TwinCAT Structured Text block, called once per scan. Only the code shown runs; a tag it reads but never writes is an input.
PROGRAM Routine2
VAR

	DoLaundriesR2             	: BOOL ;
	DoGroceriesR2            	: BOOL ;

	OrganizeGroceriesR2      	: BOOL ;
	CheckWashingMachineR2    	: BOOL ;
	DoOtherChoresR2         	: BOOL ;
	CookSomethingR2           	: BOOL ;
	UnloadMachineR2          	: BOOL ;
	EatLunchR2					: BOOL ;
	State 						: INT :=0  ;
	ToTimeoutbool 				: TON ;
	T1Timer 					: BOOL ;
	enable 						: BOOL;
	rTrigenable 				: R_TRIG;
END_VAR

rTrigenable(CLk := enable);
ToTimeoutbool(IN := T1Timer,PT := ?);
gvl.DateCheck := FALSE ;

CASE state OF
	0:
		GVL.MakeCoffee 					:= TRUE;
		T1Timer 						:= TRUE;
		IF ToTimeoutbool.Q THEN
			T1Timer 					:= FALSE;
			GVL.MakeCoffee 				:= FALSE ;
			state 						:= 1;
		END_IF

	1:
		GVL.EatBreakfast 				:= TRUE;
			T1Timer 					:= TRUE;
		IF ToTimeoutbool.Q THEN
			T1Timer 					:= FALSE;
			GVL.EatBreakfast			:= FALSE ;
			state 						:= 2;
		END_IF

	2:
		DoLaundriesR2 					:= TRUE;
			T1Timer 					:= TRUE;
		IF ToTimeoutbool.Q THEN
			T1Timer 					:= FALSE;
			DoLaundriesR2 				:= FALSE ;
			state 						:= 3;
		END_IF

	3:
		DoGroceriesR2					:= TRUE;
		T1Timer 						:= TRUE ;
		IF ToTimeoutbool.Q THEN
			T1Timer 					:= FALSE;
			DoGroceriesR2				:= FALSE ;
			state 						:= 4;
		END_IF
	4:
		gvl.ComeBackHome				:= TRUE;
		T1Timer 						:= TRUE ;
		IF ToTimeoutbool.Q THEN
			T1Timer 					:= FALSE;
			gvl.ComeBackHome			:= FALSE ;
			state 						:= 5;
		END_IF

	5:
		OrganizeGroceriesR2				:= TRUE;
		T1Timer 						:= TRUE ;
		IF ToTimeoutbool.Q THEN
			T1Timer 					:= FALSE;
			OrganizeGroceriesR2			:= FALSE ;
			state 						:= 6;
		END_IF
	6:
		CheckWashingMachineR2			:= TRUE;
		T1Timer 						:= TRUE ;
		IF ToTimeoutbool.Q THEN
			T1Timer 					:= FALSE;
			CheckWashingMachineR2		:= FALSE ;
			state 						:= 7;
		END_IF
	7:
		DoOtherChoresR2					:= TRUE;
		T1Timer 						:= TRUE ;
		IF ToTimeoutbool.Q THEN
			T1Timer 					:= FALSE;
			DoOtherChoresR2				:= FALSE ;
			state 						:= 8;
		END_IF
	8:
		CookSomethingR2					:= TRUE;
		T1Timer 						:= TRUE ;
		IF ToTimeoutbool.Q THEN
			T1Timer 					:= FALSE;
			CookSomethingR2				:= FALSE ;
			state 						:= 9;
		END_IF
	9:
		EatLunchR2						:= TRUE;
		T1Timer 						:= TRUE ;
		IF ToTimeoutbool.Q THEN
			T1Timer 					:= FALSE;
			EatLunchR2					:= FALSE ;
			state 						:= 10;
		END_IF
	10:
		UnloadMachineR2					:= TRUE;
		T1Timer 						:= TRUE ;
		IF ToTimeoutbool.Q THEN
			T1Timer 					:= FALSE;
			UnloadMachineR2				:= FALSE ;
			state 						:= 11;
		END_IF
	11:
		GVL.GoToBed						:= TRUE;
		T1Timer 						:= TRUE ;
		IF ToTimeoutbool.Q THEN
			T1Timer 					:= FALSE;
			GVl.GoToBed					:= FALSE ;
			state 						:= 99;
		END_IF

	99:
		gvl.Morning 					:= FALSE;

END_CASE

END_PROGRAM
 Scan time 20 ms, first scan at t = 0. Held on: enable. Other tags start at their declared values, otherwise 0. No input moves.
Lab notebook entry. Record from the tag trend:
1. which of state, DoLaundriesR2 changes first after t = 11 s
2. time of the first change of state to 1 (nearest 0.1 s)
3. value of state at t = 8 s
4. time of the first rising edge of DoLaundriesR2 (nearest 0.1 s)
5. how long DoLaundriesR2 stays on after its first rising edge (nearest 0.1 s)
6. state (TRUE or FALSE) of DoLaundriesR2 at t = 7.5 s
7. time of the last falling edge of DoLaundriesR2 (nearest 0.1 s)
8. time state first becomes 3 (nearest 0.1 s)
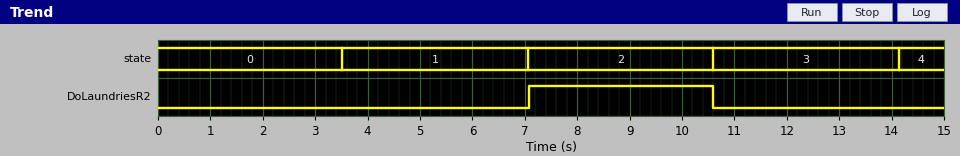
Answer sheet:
state
3.5 s
2
7.1 s
3.5 s
TRUE
10.6 s
10.6 s
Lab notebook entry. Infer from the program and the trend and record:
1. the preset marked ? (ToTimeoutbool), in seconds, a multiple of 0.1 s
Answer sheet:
3.5 s
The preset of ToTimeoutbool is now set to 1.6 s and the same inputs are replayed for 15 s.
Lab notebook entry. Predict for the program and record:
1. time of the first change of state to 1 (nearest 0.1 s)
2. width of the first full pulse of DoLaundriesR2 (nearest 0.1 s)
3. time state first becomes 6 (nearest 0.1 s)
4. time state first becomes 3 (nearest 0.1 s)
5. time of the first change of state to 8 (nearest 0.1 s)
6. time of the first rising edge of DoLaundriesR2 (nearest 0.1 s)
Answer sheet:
1.6 s
1.6 s
9.8 s
4.9 s
13.1 s
3.3 s
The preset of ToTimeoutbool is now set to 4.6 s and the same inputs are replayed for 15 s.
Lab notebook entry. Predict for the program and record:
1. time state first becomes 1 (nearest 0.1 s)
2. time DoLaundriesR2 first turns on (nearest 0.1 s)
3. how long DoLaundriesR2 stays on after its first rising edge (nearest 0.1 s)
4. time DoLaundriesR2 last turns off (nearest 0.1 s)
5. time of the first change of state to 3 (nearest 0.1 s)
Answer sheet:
4.6 s
9.3 s
4.6 s
13.9 s
13.9 s
